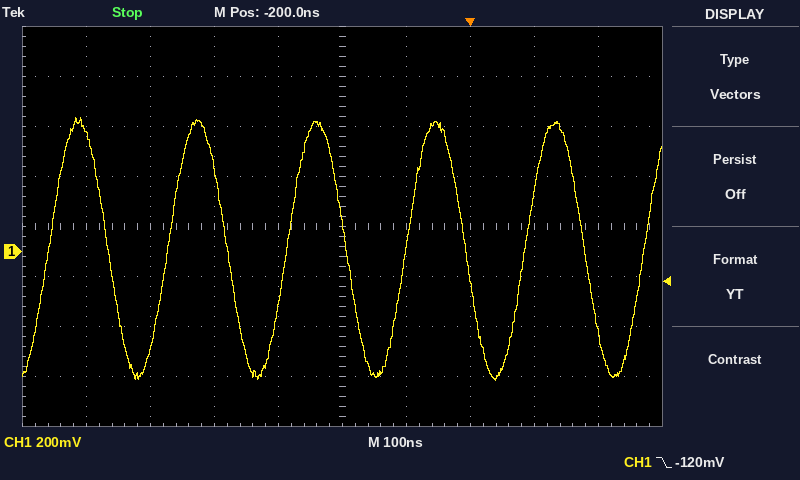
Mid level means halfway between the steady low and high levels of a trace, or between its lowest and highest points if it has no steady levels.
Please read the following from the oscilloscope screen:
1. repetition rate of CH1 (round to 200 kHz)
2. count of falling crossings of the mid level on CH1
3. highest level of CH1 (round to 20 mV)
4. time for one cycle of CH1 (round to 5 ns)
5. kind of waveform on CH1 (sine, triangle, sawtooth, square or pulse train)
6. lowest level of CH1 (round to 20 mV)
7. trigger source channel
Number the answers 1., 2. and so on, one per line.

1. 5.4 MHz
2. 5
3. 540 mV
4. 185 ns
5. sine
6. -520 mV
7. CH1
